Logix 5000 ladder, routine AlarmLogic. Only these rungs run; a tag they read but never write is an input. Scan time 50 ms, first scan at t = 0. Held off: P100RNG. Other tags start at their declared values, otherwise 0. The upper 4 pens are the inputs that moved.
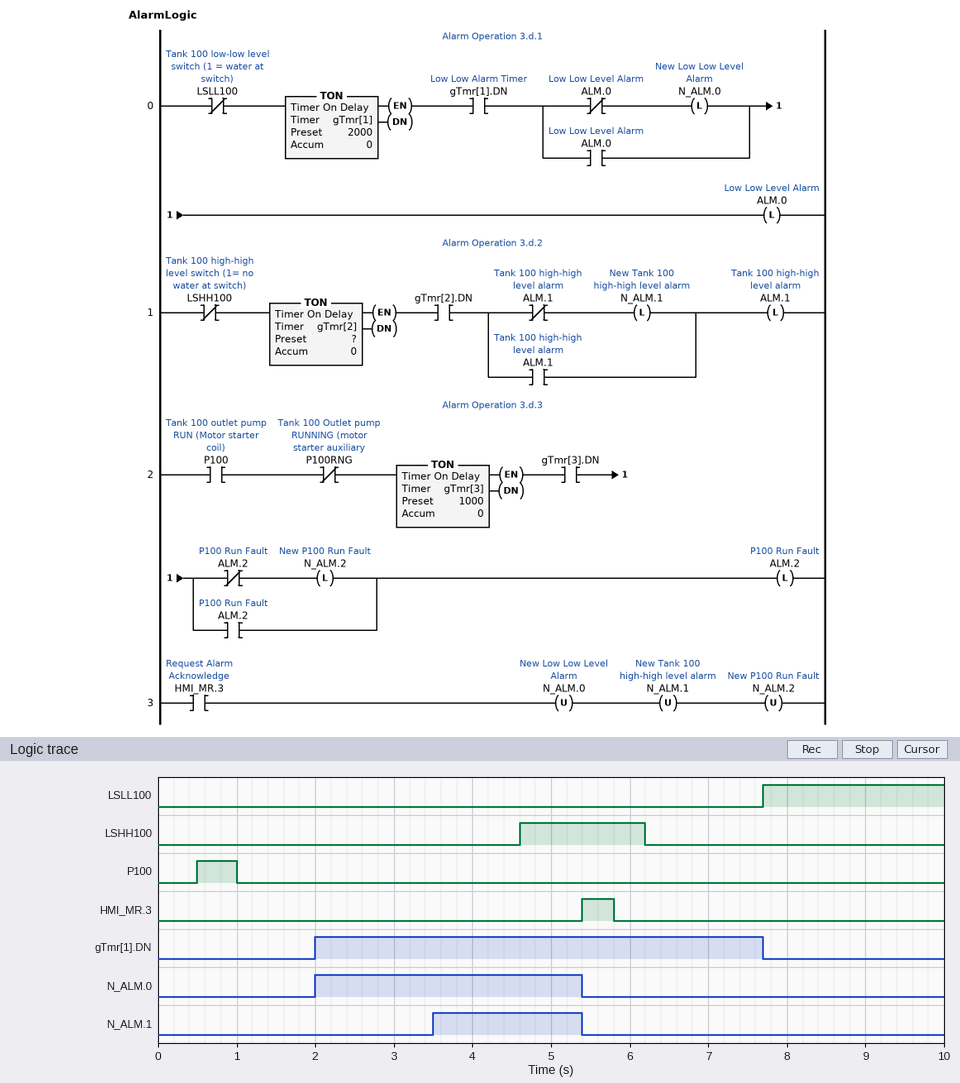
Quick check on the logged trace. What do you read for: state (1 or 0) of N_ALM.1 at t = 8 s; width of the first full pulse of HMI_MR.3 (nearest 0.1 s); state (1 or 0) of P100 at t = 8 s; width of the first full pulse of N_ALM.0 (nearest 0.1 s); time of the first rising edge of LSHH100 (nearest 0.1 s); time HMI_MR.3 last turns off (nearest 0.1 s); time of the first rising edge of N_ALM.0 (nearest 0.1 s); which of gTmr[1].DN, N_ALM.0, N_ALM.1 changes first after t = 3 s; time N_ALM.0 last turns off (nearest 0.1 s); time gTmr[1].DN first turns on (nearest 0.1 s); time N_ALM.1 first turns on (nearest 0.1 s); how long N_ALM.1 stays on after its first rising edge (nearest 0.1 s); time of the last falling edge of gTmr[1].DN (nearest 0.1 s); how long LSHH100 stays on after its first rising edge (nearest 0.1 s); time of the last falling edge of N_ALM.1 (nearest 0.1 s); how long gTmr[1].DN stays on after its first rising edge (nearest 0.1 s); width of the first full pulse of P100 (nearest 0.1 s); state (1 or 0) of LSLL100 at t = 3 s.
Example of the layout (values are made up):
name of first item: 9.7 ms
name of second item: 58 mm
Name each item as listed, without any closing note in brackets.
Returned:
state (1 or 0) of N_ALM.1 at t = 8 s: 0
width of the first full pulse of HMI_MR.3: 0.4 s
state (1 or 0) of P100 at t = 8 s: 0
width of the first full pulse of N_ALM.0: 3.4 s
time of the first rising edge of LSHH100: 4.6 s
time HMI_MR.3 last turns off: 5.8 s
time of the first rising edge of N_ALM.0: 2.0 s
which of gTmr[1].DN, N_ALM.0, N_ALM.1 changes first after t = 3 s: N_ALM.1
time N_ALM.0 last turns off: 5.4 s
time gTmr[1].DN first turns on: 2.0 s
time N_ALM.1 first turns on: 3.5 s
how long N_ALM.1 stays on after its first rising edge: 1.9 s
time of the last falling edge of gTmr[1].DN: 7.7 s
how long LSHH100 stays on after its first rising edge: 1.6 s
time of the last falling edge of N_ALM.1: 5.4 s
how long gTmr[1].DN stays on after its first rising edge: 5.7 s
width of the first full pulse of P100: 0.5 s
state (1 or 0) of LSLL100 at t = 3 s: 0
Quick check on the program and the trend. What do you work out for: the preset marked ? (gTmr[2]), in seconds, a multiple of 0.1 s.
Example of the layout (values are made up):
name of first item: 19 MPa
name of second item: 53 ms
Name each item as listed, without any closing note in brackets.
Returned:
the preset marked ? (gTmr[2]), in seconds, a multiple of 0.1 s: 3.5 s
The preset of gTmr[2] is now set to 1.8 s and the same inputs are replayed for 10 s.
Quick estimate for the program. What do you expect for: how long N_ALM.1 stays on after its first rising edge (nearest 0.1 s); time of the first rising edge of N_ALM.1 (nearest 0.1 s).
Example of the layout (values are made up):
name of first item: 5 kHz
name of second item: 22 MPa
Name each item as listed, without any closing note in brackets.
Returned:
how long N_ALM.1 stays on after its first rising edge: 3.6 s
time of the first rising edge of N_ALM.1: 1.8 s
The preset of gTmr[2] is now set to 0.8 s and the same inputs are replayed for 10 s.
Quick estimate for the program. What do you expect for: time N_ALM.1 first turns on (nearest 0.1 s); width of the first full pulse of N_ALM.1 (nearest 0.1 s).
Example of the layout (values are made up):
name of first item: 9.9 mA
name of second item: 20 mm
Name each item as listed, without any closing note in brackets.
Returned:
time N_ALM.1 first turns on: 0.8 s
width of the first full pulse of N_ALM.1: 4.6 s
